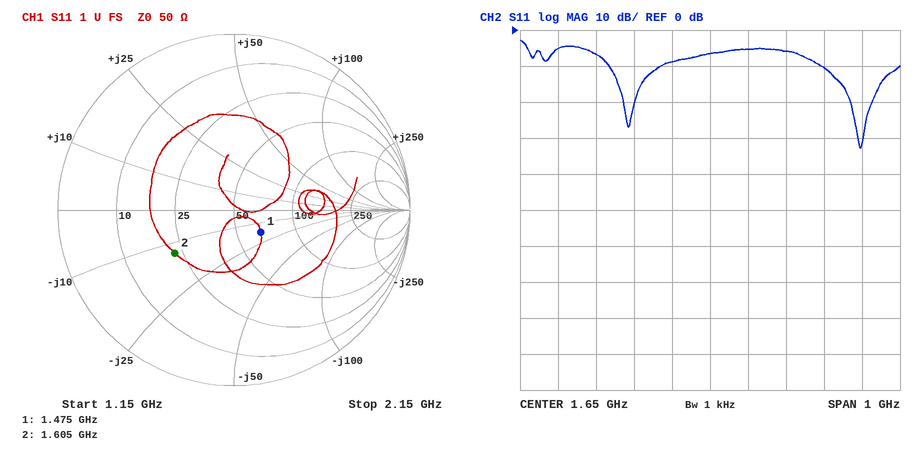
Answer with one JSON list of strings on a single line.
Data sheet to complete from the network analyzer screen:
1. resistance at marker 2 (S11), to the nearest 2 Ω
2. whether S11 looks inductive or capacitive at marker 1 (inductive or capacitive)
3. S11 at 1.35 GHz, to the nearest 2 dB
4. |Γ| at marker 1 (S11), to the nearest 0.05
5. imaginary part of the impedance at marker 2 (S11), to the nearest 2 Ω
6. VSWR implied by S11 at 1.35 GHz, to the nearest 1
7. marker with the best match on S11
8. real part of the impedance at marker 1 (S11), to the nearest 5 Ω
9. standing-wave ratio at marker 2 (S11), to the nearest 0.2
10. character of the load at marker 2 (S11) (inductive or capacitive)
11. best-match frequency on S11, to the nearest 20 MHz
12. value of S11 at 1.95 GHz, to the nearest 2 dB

["22 Ω", "capacitive", "-6 dB", "0.20", "-14 Ω", "3", "marker 1", "65 Ω", "2.4", "capacitive", "2.04 GHz", "-10 dB"]
